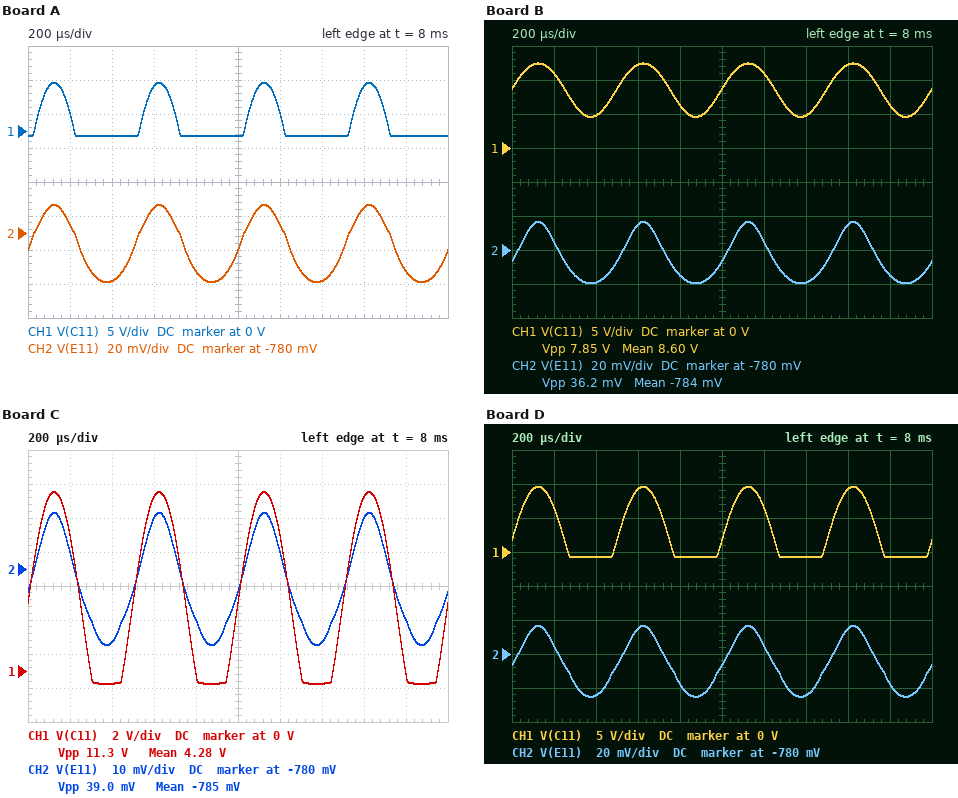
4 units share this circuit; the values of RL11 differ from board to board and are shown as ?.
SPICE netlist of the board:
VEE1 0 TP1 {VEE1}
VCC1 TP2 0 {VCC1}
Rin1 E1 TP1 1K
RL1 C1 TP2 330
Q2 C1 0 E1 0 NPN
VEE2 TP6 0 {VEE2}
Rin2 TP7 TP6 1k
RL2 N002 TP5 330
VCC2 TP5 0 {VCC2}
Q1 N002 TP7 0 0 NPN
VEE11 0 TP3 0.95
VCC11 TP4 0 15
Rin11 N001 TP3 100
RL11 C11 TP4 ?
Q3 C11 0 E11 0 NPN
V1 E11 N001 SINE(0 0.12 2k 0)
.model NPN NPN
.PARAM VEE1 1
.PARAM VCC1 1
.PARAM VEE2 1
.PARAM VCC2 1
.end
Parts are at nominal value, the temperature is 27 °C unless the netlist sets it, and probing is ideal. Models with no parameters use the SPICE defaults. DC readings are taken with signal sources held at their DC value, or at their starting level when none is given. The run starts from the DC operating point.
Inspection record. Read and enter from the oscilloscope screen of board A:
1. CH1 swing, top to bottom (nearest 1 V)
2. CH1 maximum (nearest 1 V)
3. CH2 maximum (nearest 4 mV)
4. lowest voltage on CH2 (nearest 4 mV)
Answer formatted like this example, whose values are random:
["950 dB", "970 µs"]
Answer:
["8 V", "7 V", "-764 mV", "-808 mV"]
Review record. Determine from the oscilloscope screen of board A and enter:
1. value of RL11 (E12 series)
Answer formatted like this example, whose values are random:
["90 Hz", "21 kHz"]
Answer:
["12 kΩ"]
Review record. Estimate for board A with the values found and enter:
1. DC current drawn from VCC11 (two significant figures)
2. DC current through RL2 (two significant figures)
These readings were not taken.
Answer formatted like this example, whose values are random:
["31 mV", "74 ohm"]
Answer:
["1.3 mA", "2.8 mA"]
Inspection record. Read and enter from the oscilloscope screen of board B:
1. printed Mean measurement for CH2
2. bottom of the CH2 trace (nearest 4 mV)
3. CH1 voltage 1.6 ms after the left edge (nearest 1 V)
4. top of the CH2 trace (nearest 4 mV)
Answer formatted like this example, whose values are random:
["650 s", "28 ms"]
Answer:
["-784 mV", "-800 mV", "12 V", "-764 mV"]
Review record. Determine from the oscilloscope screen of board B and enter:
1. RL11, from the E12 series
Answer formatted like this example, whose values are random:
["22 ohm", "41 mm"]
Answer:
["3.9 kΩ"]
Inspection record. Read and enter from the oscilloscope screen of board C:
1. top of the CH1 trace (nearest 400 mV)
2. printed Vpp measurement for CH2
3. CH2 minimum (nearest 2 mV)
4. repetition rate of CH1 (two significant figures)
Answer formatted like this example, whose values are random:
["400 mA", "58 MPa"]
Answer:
["10.4 V", "39.0 mV", "-802 mV", "2.0 kHz"]
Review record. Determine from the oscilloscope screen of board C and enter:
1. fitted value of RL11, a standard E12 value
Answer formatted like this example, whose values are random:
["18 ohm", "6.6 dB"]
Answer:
["6.8 kΩ"]
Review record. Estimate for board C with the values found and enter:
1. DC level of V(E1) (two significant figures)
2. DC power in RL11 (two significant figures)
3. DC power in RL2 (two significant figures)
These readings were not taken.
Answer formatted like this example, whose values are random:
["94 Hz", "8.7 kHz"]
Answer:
["-740 mV", "18 mW", "2.6 mW"]
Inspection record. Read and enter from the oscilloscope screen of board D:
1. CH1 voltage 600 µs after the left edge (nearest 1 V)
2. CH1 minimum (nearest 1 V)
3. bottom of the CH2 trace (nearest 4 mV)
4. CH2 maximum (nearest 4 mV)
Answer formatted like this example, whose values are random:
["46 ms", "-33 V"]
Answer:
["9 V", "-1 V", "-804 mV", "-764 mV"]
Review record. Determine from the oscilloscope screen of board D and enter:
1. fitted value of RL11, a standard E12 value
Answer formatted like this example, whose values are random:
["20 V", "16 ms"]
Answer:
["8.2 kΩ"]
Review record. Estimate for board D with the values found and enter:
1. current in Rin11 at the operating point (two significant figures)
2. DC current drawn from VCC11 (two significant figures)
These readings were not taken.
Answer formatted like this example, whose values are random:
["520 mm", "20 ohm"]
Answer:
["1.6 mA", "1.6 mA"]
